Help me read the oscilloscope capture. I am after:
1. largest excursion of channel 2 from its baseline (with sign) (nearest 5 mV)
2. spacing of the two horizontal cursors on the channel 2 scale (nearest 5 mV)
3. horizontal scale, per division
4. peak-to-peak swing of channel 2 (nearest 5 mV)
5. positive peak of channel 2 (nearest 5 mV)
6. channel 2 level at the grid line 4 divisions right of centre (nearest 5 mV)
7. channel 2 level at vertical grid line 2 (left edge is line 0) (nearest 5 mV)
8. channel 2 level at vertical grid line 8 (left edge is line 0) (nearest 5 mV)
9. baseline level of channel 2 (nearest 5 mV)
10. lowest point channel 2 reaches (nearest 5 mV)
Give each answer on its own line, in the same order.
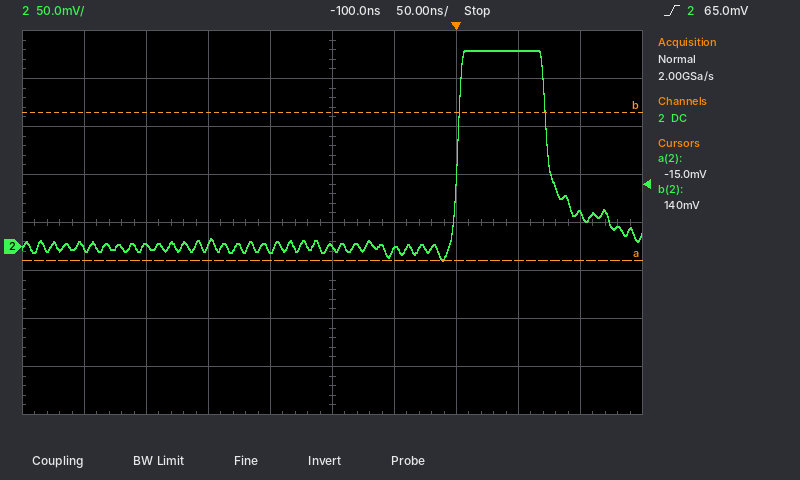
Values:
+205 mV
155 mV
50 ns
220 mV
205 mV
35 mV
0 mV
205 mV
0 mV
-15 mV
